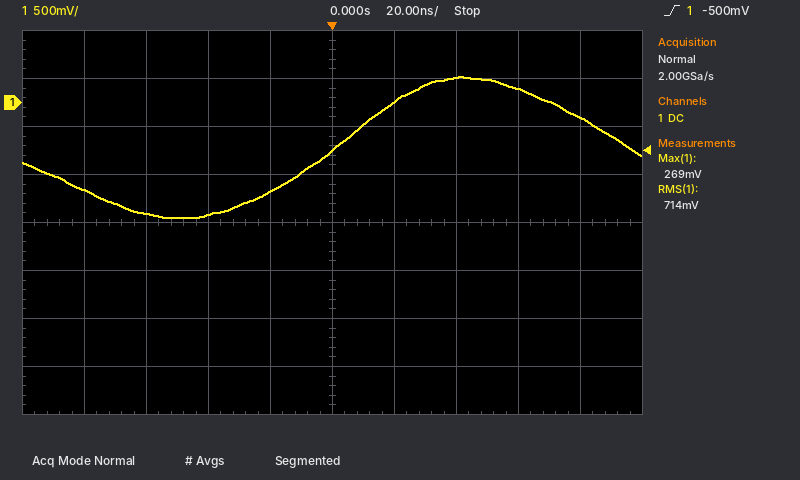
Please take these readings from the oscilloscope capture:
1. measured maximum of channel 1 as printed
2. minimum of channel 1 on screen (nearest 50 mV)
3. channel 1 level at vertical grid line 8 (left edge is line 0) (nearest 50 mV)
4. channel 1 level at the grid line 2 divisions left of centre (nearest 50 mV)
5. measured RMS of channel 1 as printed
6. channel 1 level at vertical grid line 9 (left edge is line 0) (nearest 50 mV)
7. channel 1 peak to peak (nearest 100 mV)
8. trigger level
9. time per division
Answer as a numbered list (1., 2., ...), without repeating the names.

1. 269 mV
2. -1.20 V
3. 150 mV
4. -1.15 V
5. 714 mV
6. -150 mV
7. 1.50 V
8. -500 mV
9. 20 ns
